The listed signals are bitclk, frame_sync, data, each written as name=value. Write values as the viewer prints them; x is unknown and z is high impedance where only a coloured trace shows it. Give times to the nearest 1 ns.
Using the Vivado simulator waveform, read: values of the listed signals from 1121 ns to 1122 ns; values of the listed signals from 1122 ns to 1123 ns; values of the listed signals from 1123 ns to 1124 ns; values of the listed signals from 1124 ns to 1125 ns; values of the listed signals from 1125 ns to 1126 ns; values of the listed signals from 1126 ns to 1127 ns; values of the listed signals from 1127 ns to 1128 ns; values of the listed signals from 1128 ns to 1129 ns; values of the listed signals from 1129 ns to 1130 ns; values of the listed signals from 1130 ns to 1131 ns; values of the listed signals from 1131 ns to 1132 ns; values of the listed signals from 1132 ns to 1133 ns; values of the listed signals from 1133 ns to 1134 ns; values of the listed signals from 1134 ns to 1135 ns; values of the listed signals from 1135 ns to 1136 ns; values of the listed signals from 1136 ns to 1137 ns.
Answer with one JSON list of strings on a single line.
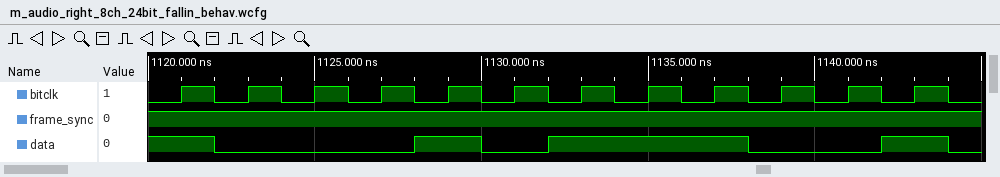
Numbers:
["bitclk=1, frame_sync=1, data=1", "bitclk=0, frame_sync=1, data=0", "bitclk=1, frame_sync=1, data=0", "bitclk=0, frame_sync=1, data=0", "bitclk=1, frame_sync=1, data=0", "bitclk=0, frame_sync=1, data=0", "bitclk=1, frame_sync=1, data=0", "bitclk=0, frame_sync=1, data=1", "bitclk=1, frame_sync=1, data=1", "bitclk=0, frame_sync=1, data=0", "bitclk=1, frame_sync=1, data=0", "bitclk=0, frame_sync=1, data=1", "bitclk=1, frame_sync=1, data=1", "bitclk=0, frame_sync=1, data=1", "bitclk=1, frame_sync=1, data=1", "bitclk=0, frame_sync=1, data=1"]
